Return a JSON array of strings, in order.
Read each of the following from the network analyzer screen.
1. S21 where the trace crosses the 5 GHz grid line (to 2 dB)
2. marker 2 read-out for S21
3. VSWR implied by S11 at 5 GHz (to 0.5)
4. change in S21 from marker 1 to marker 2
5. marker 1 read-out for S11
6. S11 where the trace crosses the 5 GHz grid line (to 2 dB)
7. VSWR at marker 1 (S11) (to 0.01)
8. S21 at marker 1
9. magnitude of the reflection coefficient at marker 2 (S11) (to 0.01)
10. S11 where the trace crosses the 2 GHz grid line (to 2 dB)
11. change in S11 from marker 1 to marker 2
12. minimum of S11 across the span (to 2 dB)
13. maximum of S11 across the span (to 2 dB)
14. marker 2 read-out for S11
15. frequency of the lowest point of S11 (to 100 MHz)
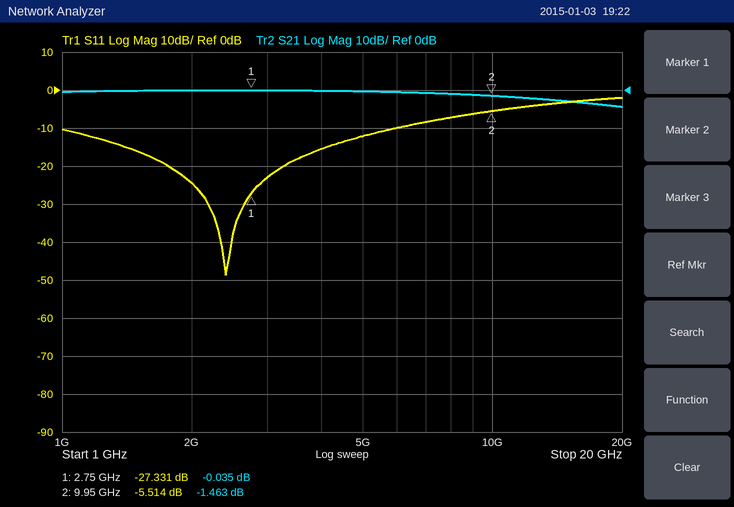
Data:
["0 dB", "-1.463 dB", "1.5", "-1.428 dB", "-27.331 dB", "-12 dB", "1.09", "-0.035 dB", "0.53", "-24 dB", "21.817 dB", "-48 dB", "-2 dB", "-5.514 dB", "2.4 GHz"]
